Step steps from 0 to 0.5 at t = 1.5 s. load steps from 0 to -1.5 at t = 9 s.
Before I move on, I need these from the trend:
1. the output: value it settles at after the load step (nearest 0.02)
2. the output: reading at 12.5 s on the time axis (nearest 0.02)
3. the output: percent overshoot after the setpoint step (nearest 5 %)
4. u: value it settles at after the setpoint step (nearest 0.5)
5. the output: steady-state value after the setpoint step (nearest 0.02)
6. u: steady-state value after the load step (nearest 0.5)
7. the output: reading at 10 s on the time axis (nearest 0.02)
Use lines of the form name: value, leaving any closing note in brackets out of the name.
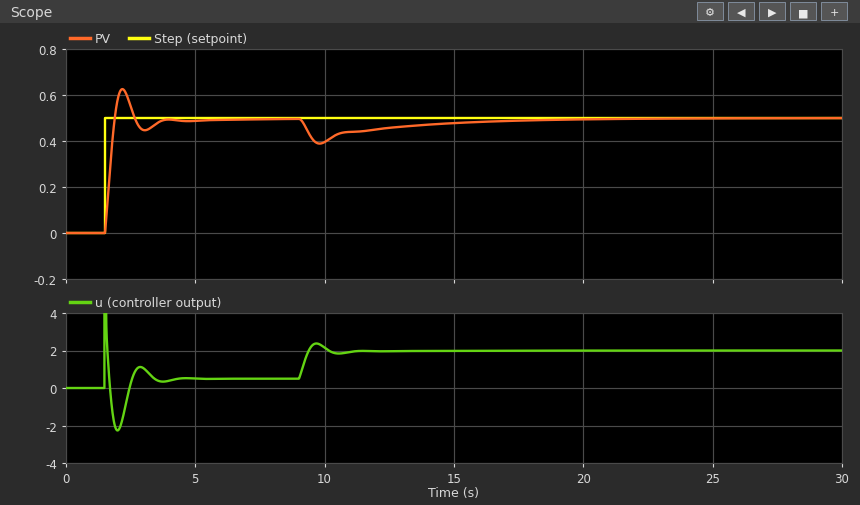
the output: value it settles at after the load step: 0.50
the output: reading at 12.5 s on the time axis: 0.46
the output: percent overshoot after the setpoint step: 25 %
u: value it settles at after the setpoint step: 0.5
the output: steady-state value after the setpoint step: 0.50
u: steady-state value after the load step: 2.0
the output: reading at 10 s on the time axis: 0.40
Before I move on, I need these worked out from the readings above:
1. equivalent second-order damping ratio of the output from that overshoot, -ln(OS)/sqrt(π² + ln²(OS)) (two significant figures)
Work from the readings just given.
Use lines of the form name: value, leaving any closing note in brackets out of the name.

equivalent second-order damping ratio of the output from that overshoot, -ln(OS)/sqrt(π² + ln²(OS)): 0.40
